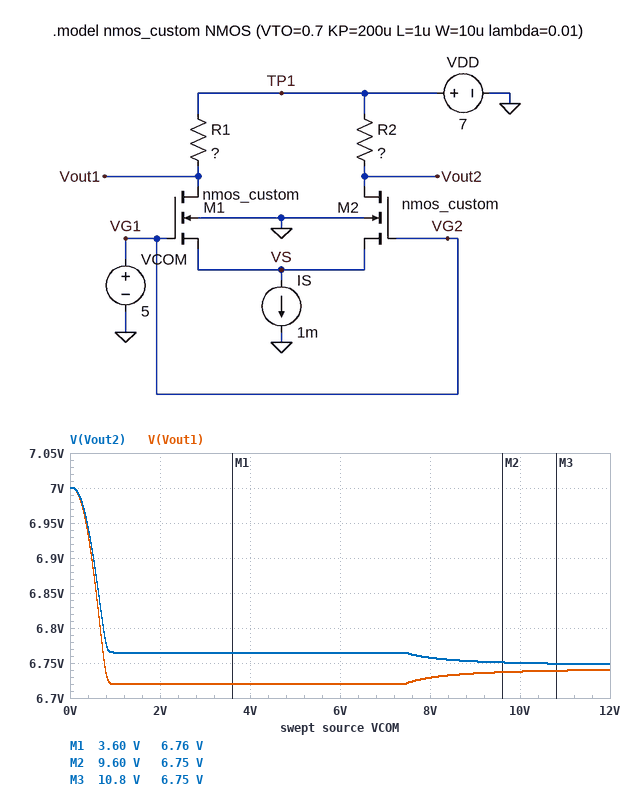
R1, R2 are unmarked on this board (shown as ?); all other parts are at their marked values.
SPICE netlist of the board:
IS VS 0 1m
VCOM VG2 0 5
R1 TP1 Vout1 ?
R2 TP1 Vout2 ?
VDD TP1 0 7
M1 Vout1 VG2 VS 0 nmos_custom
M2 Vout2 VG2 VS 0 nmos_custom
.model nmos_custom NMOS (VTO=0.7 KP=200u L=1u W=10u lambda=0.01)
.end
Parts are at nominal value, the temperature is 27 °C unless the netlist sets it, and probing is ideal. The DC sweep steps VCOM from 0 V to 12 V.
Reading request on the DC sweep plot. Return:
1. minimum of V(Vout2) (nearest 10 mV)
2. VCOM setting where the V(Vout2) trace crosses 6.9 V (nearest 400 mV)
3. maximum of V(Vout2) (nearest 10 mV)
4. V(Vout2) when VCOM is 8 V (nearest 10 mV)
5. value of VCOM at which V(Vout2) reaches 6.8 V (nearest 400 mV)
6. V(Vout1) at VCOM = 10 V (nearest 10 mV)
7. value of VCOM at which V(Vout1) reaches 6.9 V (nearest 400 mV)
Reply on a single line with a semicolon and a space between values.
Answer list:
6.75 V; 400 mV; 7.00 V; 6.76 V; 800 mV; 6.74 V; 400 mV
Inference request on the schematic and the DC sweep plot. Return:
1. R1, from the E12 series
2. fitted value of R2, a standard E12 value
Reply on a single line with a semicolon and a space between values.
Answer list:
560 Ω; 470 Ω
